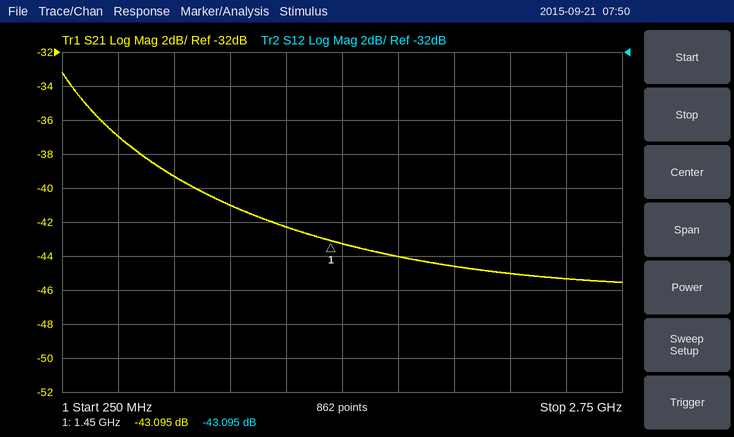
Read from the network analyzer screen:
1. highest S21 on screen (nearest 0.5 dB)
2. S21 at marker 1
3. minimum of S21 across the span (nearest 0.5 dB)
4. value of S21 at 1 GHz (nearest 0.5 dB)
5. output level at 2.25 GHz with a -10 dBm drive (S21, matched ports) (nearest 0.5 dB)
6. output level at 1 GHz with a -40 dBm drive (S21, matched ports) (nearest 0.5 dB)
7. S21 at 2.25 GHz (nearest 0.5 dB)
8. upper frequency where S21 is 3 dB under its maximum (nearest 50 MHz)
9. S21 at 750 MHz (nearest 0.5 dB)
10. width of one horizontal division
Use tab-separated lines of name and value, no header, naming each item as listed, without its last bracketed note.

highest S21 on screen	-33.0 dB
S21 at marker 1	-43.095 dB
minimum of S21 across the span	-45.5 dB
value of S21 at 1 GHz	-41.0 dB
output level at 2.25 GHz with a -10 dBm drive (S21, matched ports)	-55.0 dBm
output level at 1 GHz with a -40 dBm drive (S21, matched ports)	-81.0 dBm
S21 at 2.25 GHz	-45.0 dB
upper frequency where S21 is 3 dB under its maximum	450 MHz
S21 at 750 MHz	-39.5 dB
width of one horizontal division	250 MHz
